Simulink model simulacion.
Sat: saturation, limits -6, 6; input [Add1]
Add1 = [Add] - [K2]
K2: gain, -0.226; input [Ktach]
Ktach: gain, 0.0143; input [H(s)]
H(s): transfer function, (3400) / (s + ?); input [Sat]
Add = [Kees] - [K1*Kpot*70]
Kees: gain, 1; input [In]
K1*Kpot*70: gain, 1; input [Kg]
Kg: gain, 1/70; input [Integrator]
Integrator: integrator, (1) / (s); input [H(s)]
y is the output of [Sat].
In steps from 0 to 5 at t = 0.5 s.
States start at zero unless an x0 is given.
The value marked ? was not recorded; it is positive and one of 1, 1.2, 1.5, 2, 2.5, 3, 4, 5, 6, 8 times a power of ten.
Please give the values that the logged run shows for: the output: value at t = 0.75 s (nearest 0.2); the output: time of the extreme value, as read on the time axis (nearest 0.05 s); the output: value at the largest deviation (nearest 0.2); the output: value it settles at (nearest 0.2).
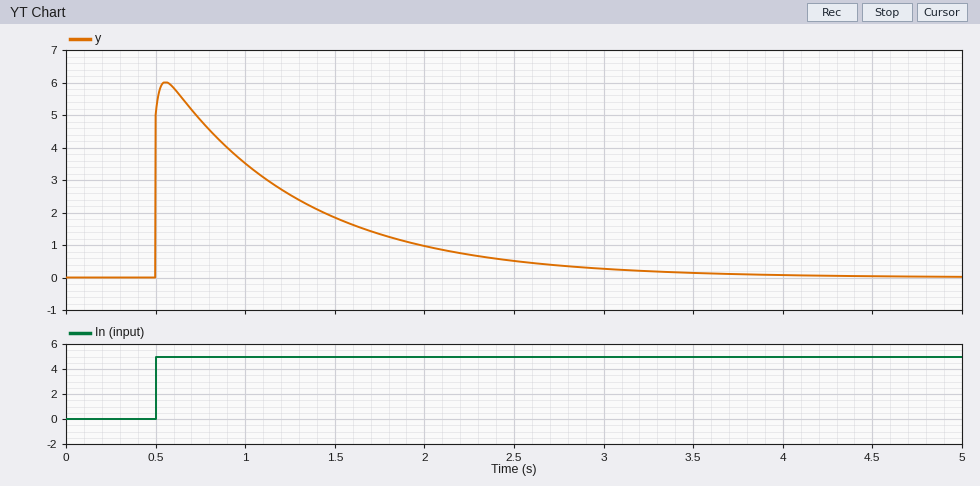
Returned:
4.8
0.55 s
6.0
0.0
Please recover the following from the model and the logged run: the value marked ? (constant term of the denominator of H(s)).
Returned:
50
